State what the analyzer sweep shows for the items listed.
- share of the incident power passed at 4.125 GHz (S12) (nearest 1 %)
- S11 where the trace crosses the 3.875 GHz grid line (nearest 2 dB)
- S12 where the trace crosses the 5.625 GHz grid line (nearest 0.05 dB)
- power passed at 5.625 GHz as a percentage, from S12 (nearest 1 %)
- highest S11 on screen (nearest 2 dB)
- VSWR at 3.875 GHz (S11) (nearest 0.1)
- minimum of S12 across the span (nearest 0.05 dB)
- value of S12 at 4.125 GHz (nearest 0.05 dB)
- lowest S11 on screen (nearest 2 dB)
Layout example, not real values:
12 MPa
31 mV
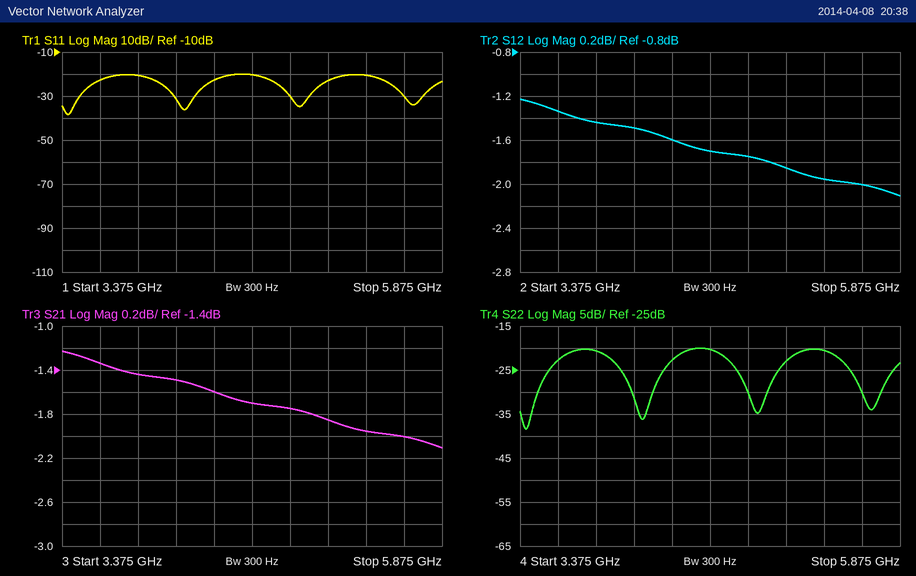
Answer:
71 %
-20 dB
-2.00 dB
63 %
-20 dB
1.2
-2.10 dB
-1.50 dB
-38 dB
